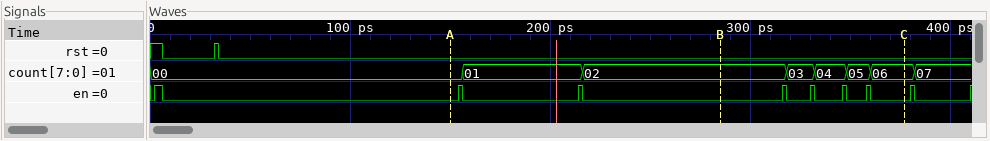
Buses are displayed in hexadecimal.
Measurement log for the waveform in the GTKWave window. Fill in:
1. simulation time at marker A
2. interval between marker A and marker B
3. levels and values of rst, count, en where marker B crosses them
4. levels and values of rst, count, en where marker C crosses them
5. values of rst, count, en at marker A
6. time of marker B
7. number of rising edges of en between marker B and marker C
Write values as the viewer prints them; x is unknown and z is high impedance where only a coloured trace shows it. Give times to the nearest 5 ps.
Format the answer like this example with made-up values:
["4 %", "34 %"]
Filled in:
["150 ps", "135 ps", "rst=0, count=02, en=0", "rst=0, count=06, en=0", "rst=0, count=00, en=0", "285 ps", "4"]
